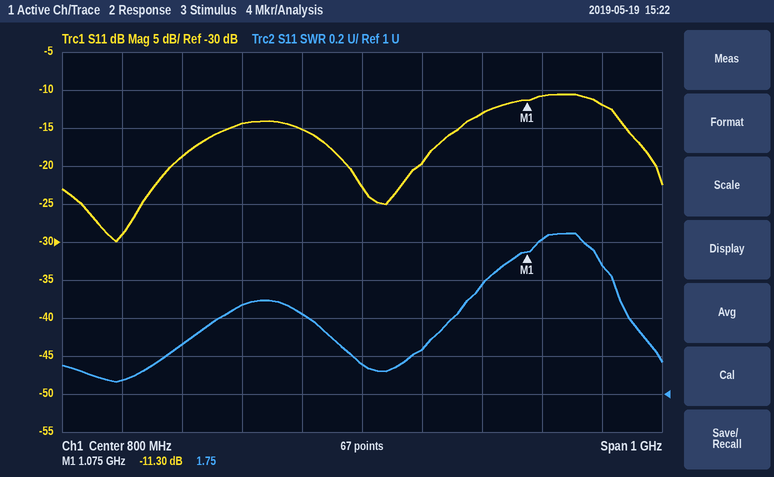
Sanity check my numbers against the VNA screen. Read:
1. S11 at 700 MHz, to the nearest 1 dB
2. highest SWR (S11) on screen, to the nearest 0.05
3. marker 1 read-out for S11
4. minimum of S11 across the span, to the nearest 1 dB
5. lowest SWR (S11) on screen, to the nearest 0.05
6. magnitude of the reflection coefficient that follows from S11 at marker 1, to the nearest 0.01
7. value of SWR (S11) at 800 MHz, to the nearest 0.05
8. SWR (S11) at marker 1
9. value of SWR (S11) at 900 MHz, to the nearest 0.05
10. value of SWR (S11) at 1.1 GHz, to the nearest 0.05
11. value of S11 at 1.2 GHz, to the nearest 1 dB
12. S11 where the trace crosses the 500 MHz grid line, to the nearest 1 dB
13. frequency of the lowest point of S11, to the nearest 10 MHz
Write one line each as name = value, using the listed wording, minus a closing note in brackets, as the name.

S11 at 700 MHz, to the nearest 1 dB = -15 dB
highest SWR (S11) on screen, to the nearest 0.05 = 1.85
marker 1 read-out for S11 = -11.30 dB
minimum of S11 across the span, to the nearest 1 dB = -30 dB
lowest SWR (S11) on screen, to the nearest 0.05 = 1.05
magnitude of the reflection coefficient that follows from S11 at marker 1, to the nearest 0.01 = 0.27
value of SWR (S11) at 800 MHz, to the nearest 0.05 = 1.15
SWR (S11) at marker 1 = 1.75
value of SWR (S11) at 900 MHz, to the nearest 0.05 = 1.25
value of SWR (S11) at 1.1 GHz, to the nearest 0.05 = 1.80
value of S11 at 1.2 GHz, to the nearest 1 dB = -12 dB
S11 where the trace crosses the 500 MHz grid line, to the nearest 1 dB = -19 dB
frequency of the lowest point of S11, to the nearest 10 MHz = 390 MHz
